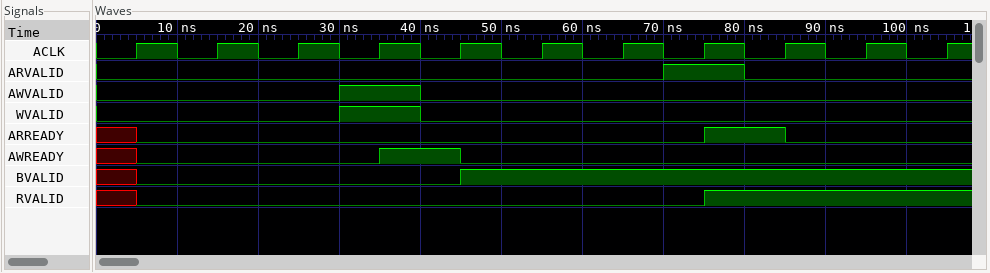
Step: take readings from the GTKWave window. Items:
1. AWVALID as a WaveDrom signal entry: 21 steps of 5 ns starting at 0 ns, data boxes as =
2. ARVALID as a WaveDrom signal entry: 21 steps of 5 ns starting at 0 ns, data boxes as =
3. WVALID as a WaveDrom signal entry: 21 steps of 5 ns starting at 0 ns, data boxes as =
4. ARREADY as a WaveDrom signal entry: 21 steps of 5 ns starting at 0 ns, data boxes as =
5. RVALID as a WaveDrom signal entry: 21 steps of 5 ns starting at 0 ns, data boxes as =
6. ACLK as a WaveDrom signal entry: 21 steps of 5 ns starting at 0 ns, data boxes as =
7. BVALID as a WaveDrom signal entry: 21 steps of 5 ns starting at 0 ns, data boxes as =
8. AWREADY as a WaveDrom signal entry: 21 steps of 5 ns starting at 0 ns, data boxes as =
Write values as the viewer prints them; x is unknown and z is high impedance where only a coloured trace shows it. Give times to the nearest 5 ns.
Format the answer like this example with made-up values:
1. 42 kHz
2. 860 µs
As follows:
1. {name: 'AWVALID', wave: '0.....1.0............'}
2. {name: 'ARVALID', wave: '0.............1.0....'}
3. {name: 'WVALID', wave: '0.....1.0............'}
4. {name: 'ARREADY', wave: 'x0.............1.0...'}
5. {name: 'RVALID', wave: 'x0.............1.....'}
6. {name: 'ACLK', wave: '010101010101010101010'}
7. {name: 'BVALID', wave: 'x0.......1...........'}
8. {name: 'AWREADY', wave: 'x0.....1.0...........'}
